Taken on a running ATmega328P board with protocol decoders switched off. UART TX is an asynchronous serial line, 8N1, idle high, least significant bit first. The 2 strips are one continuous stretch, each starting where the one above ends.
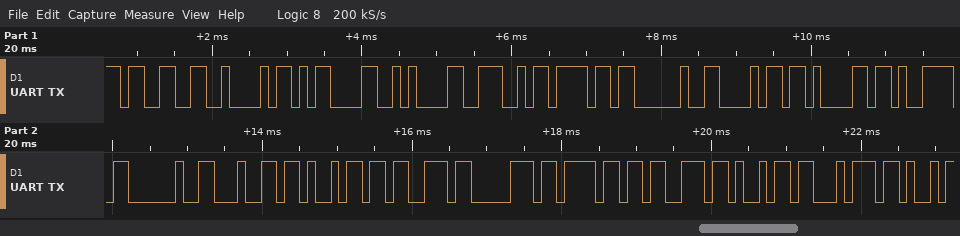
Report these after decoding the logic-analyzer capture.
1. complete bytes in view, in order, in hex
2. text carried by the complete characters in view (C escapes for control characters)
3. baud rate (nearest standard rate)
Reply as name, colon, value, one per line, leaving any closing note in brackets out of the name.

complete bytes in view, in order, in hex: 0x33 0x42 0x0D 0x0A 0x4E 0x6F 0x20 0x68 0x61 0x79 0x20 0x64 0x69 0x73 0x70 0x6F 0x73 0x69 0x74
text carried by the complete characters in view: "3B\r\nNo hay disposit"
baud rate: 9600 baud
